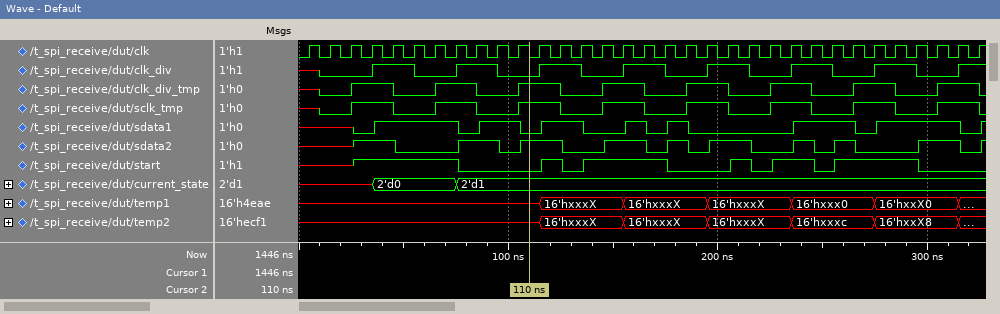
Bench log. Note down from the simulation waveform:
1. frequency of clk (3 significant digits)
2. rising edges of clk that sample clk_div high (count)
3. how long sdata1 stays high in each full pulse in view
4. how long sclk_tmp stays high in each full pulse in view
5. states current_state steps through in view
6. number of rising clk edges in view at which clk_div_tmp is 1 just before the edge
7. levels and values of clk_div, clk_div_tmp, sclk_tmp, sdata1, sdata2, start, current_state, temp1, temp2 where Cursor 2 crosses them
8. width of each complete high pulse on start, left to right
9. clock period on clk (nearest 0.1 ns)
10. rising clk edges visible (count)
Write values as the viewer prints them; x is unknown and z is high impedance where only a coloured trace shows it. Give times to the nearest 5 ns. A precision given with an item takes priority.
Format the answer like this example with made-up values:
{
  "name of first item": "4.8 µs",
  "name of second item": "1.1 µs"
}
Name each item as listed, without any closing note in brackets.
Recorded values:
{
  "frequency of clk": "100 MHz",
  "rising edges of clk that sample clk_div high": "15",
  "how long sdata1 stays high in each full pulse in view": "40 ns, 20 ns, 20 ns, 10 ns, 10 ns, 30 ns, 40 ns",
  "how long sclk_tmp stays high in each full pulse in view": "20 ns, 20 ns, 20 ns, 20 ns, 20 ns, 20 ns, 20 ns, 20 ns",
  "states current_state steps through in view": "x, 2'd0, 2'd1",
  "number of rising clk edges in view at which clk_div_tmp is 1 just before the edge": "16",
  "levels and values of clk_div, clk_div_tmp, sclk_tmp, sdata1, sdata2, start, current_state, temp1, temp2 where Cursor 2 crosses them": "clk_div=0, clk_div_tmp=1, sclk_tmp=1, sdata1=0, sdata2=1, start=0, current_state=2'd1, temp1=x, temp2=x",
  "width of each complete high pulse on start, left to right": "10 ns, 40 ns, 10 ns, 20 ns, 40 ns",
  "clock period on clk": "10 ns",
  "rising clk edges visible": "33"
}
